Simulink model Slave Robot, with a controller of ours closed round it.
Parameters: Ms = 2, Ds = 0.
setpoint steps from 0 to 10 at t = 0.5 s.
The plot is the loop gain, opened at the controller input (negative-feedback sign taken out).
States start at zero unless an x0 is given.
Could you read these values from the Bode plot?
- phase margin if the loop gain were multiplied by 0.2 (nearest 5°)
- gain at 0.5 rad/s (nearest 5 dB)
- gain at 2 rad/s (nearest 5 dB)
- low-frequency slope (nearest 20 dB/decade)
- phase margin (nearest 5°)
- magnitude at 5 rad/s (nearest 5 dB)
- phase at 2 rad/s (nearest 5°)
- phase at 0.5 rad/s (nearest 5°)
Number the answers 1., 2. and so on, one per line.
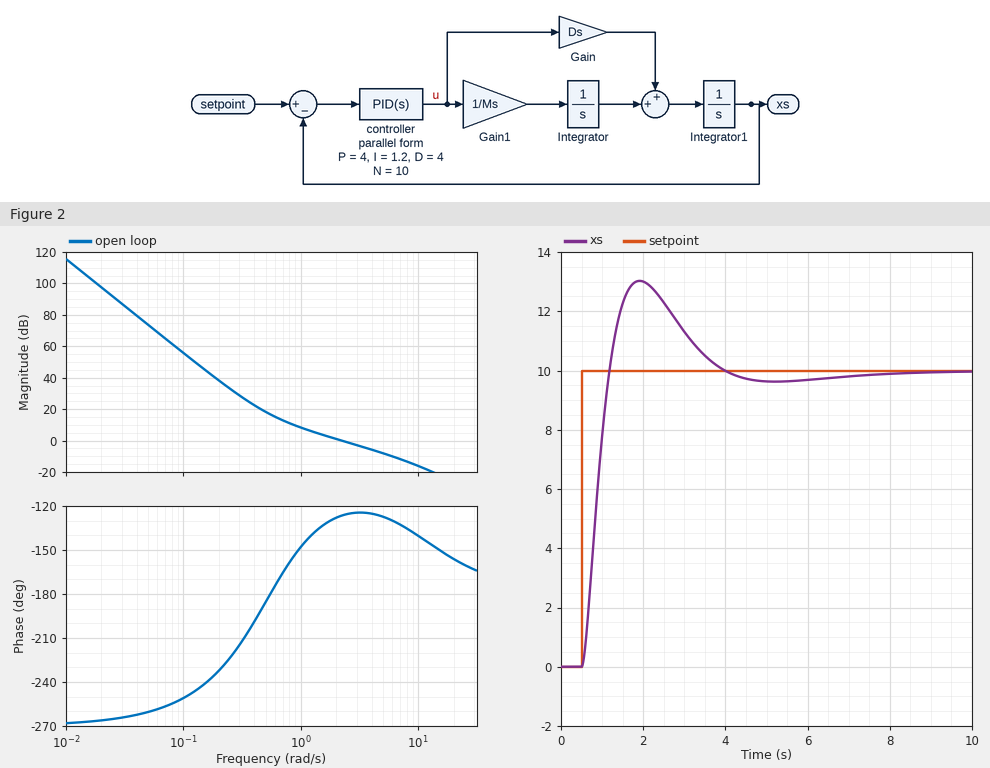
1. 10°
2. 20 dB
3. 0 dB
4. -60 dB/decade
5. 55°
6. -10 dB
7. -130°
8. -185°
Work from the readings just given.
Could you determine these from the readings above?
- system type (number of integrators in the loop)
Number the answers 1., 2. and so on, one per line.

1. 3
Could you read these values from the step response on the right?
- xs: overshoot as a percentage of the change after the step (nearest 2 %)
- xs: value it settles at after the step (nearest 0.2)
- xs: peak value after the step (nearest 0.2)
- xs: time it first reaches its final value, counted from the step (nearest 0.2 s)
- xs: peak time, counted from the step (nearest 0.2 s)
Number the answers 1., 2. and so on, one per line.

1. 30 %
2. 10.0
3. 13.0
4. 0.6 s
5. 1.4 s
